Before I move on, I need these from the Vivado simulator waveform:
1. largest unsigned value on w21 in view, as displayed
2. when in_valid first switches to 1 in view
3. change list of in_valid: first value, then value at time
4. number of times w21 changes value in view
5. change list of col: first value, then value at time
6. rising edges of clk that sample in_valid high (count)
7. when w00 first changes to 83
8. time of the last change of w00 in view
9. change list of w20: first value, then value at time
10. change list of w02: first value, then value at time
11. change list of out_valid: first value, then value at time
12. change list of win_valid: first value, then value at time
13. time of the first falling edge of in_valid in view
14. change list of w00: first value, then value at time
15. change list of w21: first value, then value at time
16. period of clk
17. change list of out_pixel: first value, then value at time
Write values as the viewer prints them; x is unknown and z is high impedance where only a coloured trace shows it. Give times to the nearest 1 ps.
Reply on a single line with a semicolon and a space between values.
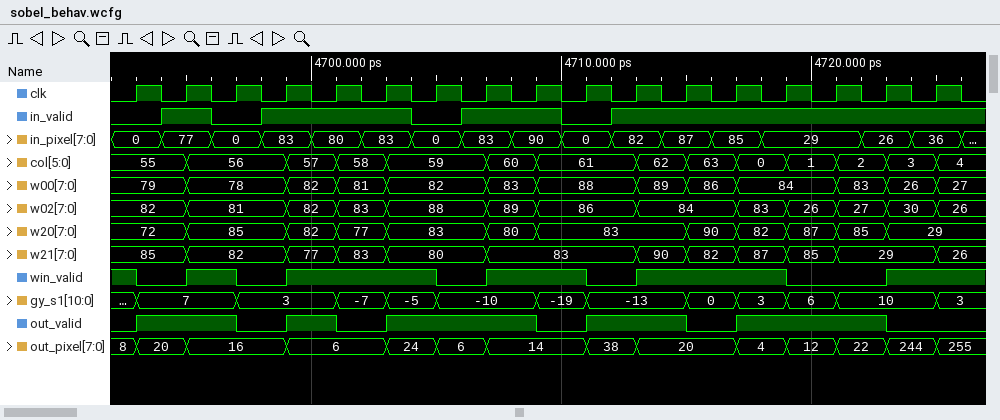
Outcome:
90; 4694 ps; 0, 1 at 4694 ps, 0 at 4696 ps, 1 at 4698 ps, 0 at 4704 ps, 1 at 4706 ps, 0 at 4710 ps, 1 at 4712 ps; 11; 55, 56 at 4695 ps, 57 at 4699 ps, 58 at 4701 ps, 59 at 4703 ps, 60 at 4707 ps, 61 at 4709 ps, 62 at 4713 ps, 63 at 4715 ps, 0 at 4717 ps, 1 at 4719 ps, 2 at 4721 ps, 3 at 4723 ps, 4 at 4725 ps; 13; 4707 ps; 4725 ps; 72, 85 at 4695 ps, 82 at 4699 ps, 77 at 4701 ps, 83 at 4703 ps, 80 at 4707 ps, 83 at 4709 ps, 90 at 4715 ps, 82 at 4717 ps, 87 at 4719 ps, 85 at 4721 ps, 29 at 4723 ps; 82, 81 at 4695 ps, 82 at 4699 ps, 83 at 4701 ps, 88 at 4703 ps, 89 at 4707 ps, 86 at 4709 ps, 84 at 4713 ps, 83 at 4717 ps, 26 at 4719 ps, 27 at 4721 ps, 30 at 4723 ps, 26 at 4725 ps; 0, 1 at 4693 ps, 0 at 4697 ps, 1 at 4699 ps, 0 at 4701 ps, 1 at 4703 ps, 0 at 4709 ps, 1 at 4711 ps, 0 at 4715 ps, 1 at 4717 ps, 0 at 4723 ps; 1, 0 at 4693 ps, 1 at 4695 ps, 0 at 4697 ps, 1 at 4699 ps, 0 at 4705 ps, 1 at 4707 ps, 0 at 4711 ps, 1 at 4713 ps, 0 at 4719 ps, 1 at 4723 ps; 4696 ps; 79, 78 at 4695 ps, 82 at 4699 ps, 81 at 4701 ps, 82 at 4703 ps, 83 at 4707 ps, 88 at 4709 ps, 89 at 4713 ps, 86 at 4715 ps, 84 at 4717 ps, 83 at 4721 ps, 26 at 4723 ps, 27 at 4725 ps; 85, 82 at 4695 ps, 77 at 4699 ps, 83 at 4701 ps, 80 at 4703 ps, 83 at 4707 ps, 90 at 4713 ps, 82 at 4715 ps, 87 at 4717 ps, 85 at 4719 ps, 29 at 4721 ps, 26 at 4725 ps; 2 ps; 8, 20 at 4693 ps, 16 at 4695 ps, 6 at 4699 ps, 24 at 4703 ps, 6 at 4705 ps, 14 at 4707 ps, 38 at 4711 ps, 20 at 4713 ps, 4 at 4717 ps, 12 at 4719 ps, 22 at 4721 ps, 244 at 4723 ps, 255 at 4725 ps
